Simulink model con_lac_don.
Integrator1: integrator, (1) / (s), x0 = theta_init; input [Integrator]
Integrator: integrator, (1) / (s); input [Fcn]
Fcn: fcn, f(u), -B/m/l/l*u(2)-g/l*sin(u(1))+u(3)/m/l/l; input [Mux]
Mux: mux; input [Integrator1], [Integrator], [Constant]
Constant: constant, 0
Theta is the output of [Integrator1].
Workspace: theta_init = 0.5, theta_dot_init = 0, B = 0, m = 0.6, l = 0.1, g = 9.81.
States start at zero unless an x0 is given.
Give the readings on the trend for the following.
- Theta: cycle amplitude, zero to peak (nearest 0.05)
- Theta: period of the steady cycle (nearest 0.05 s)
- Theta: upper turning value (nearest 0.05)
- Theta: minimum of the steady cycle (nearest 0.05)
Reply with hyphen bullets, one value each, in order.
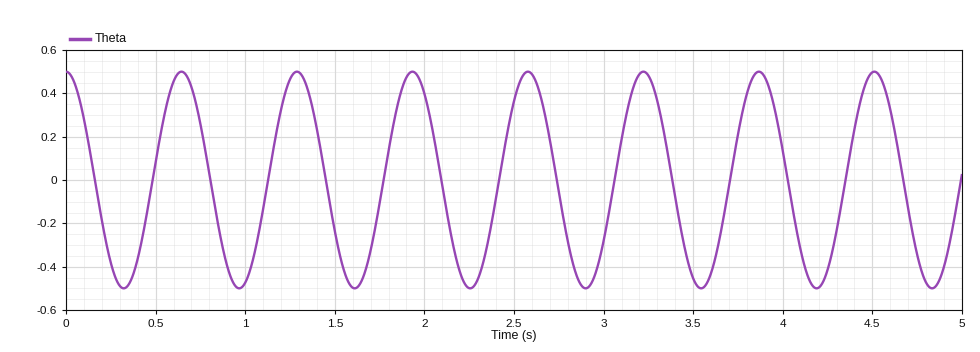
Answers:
- 0.50
- 0.65 s
- 0.50
- -0.50
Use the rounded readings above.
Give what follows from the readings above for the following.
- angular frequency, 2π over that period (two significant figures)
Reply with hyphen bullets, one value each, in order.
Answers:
- 9.7 rad/s
